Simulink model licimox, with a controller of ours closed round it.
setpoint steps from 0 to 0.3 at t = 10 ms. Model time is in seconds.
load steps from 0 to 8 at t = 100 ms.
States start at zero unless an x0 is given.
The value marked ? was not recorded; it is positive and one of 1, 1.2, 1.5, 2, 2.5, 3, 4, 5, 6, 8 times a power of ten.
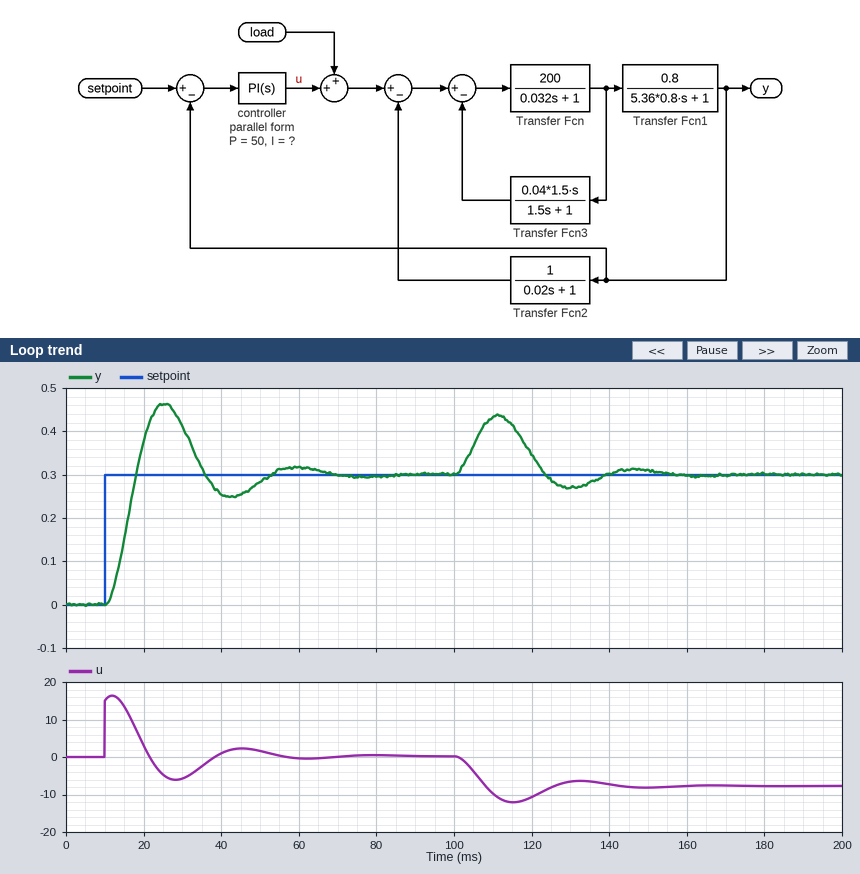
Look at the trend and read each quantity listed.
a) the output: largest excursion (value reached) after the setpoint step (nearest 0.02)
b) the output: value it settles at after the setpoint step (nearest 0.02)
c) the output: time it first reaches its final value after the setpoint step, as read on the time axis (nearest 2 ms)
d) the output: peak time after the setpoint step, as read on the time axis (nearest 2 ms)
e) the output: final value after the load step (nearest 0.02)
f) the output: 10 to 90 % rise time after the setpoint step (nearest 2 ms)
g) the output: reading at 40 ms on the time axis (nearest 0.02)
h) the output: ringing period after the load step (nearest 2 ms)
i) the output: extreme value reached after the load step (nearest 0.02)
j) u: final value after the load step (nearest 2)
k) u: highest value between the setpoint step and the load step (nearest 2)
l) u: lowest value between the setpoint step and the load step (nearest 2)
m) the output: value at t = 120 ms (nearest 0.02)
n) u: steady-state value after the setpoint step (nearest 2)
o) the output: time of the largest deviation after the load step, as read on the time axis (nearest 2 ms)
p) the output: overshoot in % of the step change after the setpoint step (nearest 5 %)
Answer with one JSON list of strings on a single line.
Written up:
["0.46", "0.30", "18 ms", "26 ms", "0.30", "6 ms", "0.26", "36 ms", "0.44", "-8", "16", "-6", "0.34", "0", "112 ms", "55 %"]
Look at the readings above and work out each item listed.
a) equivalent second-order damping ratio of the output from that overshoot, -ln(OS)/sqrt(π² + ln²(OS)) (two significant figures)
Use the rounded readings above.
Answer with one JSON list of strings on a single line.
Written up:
["0.19"]
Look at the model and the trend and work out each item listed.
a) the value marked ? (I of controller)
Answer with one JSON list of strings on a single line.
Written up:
["5000"]
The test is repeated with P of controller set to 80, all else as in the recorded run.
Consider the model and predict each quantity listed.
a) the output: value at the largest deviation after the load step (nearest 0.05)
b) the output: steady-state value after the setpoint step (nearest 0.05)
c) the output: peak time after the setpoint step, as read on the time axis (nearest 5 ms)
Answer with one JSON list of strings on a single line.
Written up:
["0.40", "0.30", "20 ms"]
